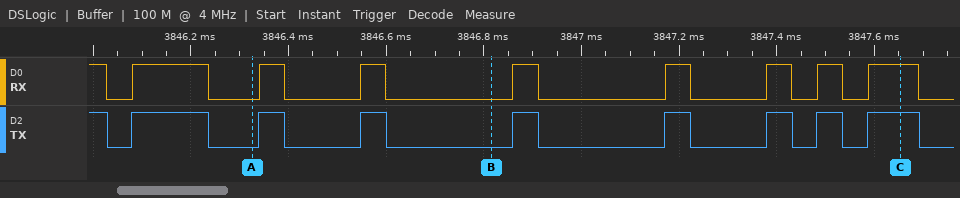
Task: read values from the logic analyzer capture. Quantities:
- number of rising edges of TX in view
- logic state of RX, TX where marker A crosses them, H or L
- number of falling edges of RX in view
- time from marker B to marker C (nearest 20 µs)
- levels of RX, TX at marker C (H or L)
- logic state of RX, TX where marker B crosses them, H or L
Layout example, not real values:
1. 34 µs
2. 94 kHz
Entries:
1. 8
2. RX=L, TX=L
3. 9
4. 840 µs
5. RX=H, TX=H
6. RX=L, TX=L
